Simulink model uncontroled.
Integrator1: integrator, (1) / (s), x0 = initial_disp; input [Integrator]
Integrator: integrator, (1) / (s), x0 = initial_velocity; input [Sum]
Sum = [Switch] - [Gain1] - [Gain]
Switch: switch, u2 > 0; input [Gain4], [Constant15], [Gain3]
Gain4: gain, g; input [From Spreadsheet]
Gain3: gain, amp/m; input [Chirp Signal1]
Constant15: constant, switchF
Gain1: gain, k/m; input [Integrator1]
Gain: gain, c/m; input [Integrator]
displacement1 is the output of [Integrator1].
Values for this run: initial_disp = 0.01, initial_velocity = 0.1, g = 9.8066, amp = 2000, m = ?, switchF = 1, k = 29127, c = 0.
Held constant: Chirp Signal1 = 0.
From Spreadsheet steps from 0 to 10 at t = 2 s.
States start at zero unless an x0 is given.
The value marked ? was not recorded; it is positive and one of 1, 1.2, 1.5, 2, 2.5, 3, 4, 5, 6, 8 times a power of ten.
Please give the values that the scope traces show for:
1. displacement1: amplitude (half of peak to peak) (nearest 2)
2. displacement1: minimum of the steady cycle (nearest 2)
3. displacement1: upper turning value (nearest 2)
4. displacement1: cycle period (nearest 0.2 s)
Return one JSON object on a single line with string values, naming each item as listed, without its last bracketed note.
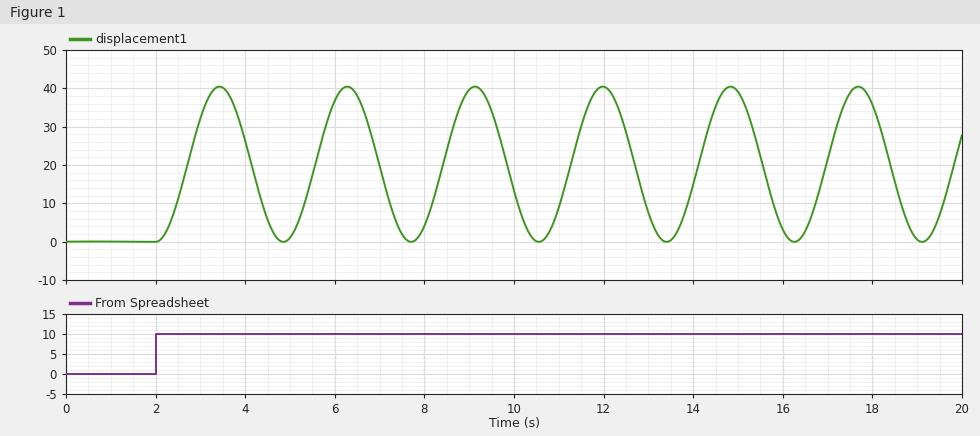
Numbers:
{"displacement1: amplitude (half of peak to peak)": "20", "displacement1: minimum of the steady cycle": "0", "displacement1: upper turning value": "40", "displacement1: cycle period": "2.8 s"}
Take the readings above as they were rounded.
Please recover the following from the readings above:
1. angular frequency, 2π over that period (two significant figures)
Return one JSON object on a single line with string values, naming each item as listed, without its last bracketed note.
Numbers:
{"angular frequency, 2π over that period": "2.2 rad/s"}
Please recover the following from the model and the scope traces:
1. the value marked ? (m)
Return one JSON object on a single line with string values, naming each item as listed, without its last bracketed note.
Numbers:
{"the value marked ?": "6000"}
